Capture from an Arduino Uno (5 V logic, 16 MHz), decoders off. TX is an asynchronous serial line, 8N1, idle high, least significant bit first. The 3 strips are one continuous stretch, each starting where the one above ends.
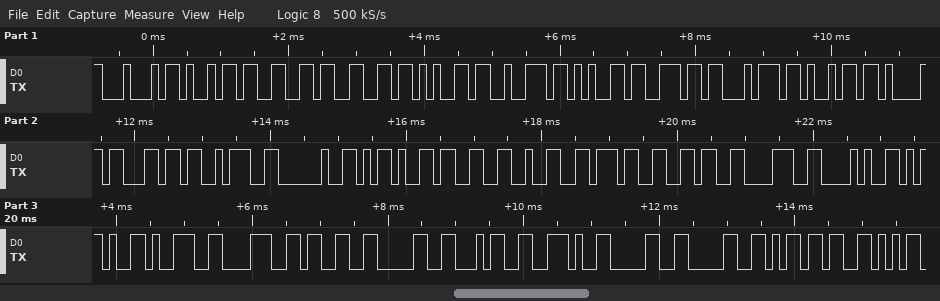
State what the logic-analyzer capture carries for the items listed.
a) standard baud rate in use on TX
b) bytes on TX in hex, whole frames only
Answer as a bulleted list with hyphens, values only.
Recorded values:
- 9600 baud
- 44 69 66 66 65 72 65 6E 74 69 61 6C 3A 20 2D 33 32 37 36 38 28 2D 39 38 33 30 34 2E 30 30 6D 56
